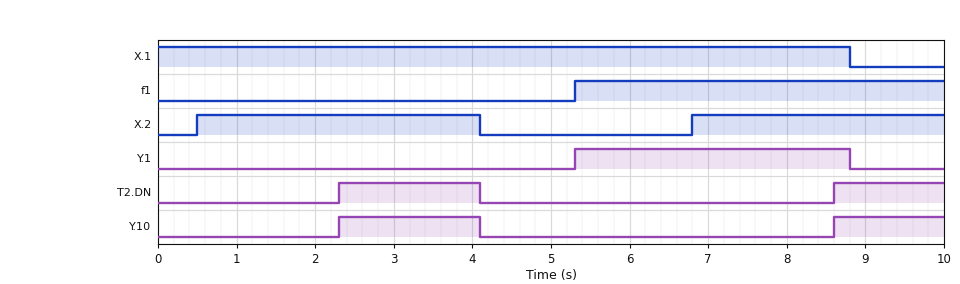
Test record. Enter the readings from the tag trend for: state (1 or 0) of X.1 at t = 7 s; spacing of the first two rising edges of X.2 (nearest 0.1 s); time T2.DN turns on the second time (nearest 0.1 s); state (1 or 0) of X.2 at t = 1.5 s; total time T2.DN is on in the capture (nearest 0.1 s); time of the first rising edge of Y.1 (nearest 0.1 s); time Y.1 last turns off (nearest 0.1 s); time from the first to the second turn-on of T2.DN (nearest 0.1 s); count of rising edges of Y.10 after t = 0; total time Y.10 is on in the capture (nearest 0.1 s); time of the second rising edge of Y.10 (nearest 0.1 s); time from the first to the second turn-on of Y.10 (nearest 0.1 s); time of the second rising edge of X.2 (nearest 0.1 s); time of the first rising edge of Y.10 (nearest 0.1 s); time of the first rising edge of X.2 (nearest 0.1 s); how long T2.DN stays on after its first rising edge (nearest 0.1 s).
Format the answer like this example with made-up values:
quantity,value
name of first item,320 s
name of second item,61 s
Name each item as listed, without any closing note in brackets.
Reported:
quantity,value
state (1 or 0) of X.1 at t = 7 s,1
spacing of the first two rising edges of X.2,6.3 s
time T2.DN turns on the second time,8.6 s
state (1 or 0) of X.2 at t = 1.5 s,1
total time T2.DN is on in the capture,3.2 s
time of the first rising edge of Y.1,5.3 s
time Y.1 last turns off,8.8 s
time from the first to the second turn-on of T2.DN,6.3 s
count of rising edges of Y.10 after t = 0,2
total time Y.10 is on in the capture,3.2 s
time of the second rising edge of Y.10,8.6 s
time from the first to the second turn-on of Y.10,6.3 s
time of the second rising edge of X.2,6.8 s
time of the first rising edge of Y.10,2.3 s
time of the first rising edge of X.2,0.5 s
how long T2.DN stays on after its first rising edge,1.8 s
